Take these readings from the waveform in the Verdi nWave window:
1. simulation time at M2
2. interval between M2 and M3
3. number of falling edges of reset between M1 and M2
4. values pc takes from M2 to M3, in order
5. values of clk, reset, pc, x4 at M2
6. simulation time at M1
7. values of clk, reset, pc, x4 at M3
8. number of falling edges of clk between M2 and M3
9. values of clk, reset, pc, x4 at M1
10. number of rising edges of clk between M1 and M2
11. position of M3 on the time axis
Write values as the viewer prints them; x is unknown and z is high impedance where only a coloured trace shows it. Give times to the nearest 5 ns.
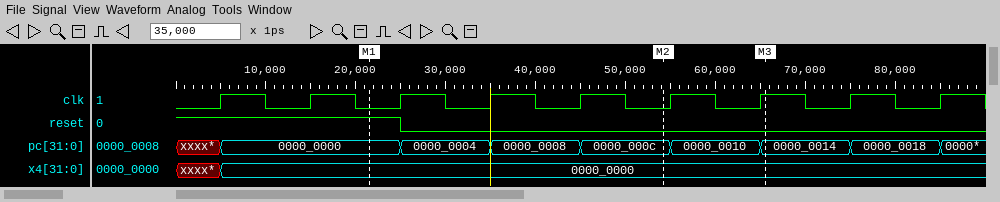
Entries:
55 ns
10 ns
1
0000_000c, 0000_0010, 0000_0014
clk=0, reset=0, pc=0000_000c, x4=0000_0000
20 ns
clk=1, reset=0, pc=0000_0014, x4=0000_0000
1
clk=0, reset=1, pc=0000_0000, x4=0000_0000
3
65 ns
